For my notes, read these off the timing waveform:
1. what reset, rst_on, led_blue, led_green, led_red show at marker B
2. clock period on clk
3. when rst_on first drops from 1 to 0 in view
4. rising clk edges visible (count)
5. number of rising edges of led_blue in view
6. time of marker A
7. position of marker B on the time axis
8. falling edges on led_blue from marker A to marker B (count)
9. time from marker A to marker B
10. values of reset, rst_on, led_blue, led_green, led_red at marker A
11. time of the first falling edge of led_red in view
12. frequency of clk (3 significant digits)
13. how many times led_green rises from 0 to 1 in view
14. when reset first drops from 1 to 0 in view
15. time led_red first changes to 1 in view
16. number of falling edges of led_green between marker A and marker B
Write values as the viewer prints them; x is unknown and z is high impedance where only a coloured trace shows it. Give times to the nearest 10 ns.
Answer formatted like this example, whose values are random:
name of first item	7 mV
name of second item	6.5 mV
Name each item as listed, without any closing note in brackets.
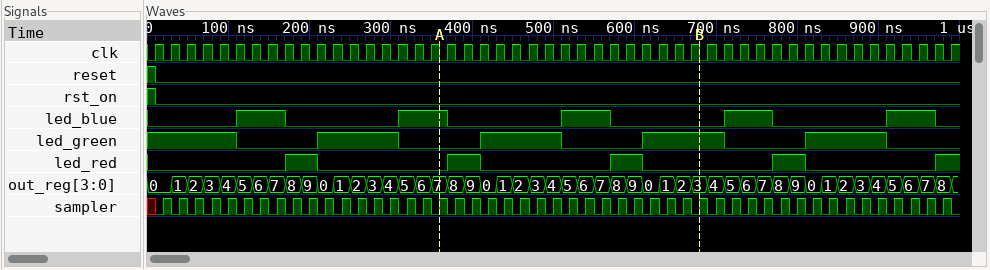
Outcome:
what reset, rst_on, led_blue, led_green, led_red show at marker B	reset=0, rst_on=0, led_blue=0, led_green=1, led_red=0
clock period on clk	20 ns
when rst_on first drops from 1 to 0 in view	10 ns
rising clk edges visible	50
number of rising edges of led_blue in view	5
time of marker A	360 ns
position of marker B on the time axis	680 ns
falling edges on led_blue from marker A to marker B	2
time from marker A to marker B	320 ns
values of reset, rst_on, led_blue, led_green, led_red at marker A	reset=0, rst_on=0, led_blue=1, led_green=0, led_red=0
time of the first falling edge of led_red in view	210 ns
frequency of clk	50.0 MHz
how many times led_green rises from 0 to 1 in view	4
when reset first drops from 1 to 0 in view	10 ns
time led_red first changes to 1 in view	170 ns
number of falling edges of led_green between marker A and marker B	1
